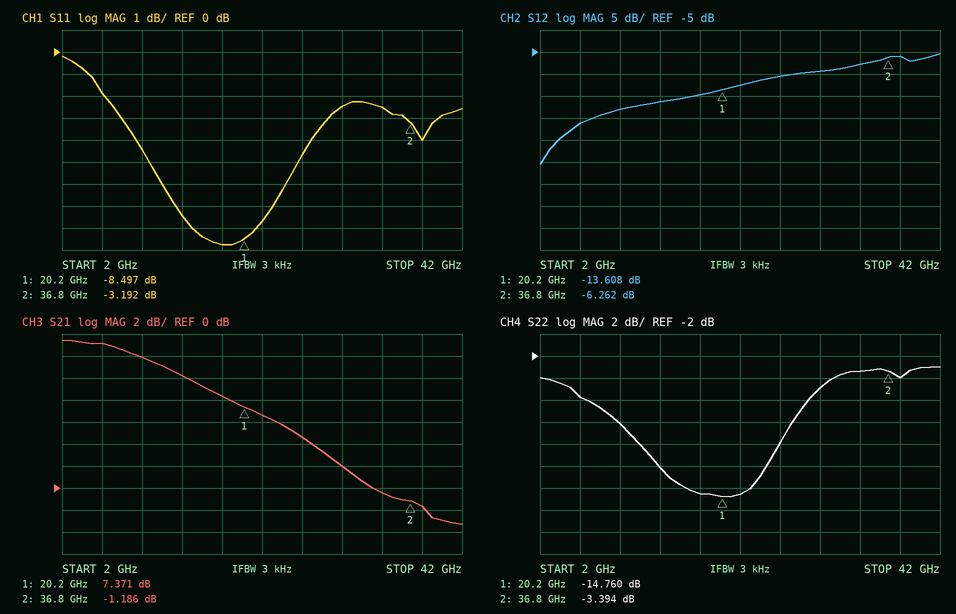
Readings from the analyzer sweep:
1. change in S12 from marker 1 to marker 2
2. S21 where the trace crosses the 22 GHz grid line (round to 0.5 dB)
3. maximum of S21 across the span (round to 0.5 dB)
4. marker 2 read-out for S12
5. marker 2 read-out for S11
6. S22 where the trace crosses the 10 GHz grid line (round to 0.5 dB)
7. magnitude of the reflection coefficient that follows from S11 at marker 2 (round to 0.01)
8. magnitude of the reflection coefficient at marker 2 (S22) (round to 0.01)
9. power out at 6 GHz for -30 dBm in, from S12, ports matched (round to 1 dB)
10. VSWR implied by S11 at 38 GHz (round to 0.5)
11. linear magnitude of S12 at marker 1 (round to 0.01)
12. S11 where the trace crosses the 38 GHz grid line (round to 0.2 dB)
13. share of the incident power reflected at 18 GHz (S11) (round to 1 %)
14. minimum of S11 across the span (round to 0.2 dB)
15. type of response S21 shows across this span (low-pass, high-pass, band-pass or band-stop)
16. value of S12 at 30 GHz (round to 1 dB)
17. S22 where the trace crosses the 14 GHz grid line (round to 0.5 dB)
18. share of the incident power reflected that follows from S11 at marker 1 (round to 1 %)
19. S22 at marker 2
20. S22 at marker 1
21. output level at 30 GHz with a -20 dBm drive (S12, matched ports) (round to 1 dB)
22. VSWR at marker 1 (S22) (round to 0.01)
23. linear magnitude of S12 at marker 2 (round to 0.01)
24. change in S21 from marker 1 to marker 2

7.346 dB
6.5 dB
13.5 dB
-6.262 dB
-3.192 dB
-8.0 dB
0.69
0.68
-51 dBm
4.5
0.21
-4.0 dB
13 %
-8.8 dB
low-pass
-9 dB
-12.0 dB
14 %
-3.394 dB
-14.760 dB
-29 dBm
1.45
0.49
-8.557 dB
